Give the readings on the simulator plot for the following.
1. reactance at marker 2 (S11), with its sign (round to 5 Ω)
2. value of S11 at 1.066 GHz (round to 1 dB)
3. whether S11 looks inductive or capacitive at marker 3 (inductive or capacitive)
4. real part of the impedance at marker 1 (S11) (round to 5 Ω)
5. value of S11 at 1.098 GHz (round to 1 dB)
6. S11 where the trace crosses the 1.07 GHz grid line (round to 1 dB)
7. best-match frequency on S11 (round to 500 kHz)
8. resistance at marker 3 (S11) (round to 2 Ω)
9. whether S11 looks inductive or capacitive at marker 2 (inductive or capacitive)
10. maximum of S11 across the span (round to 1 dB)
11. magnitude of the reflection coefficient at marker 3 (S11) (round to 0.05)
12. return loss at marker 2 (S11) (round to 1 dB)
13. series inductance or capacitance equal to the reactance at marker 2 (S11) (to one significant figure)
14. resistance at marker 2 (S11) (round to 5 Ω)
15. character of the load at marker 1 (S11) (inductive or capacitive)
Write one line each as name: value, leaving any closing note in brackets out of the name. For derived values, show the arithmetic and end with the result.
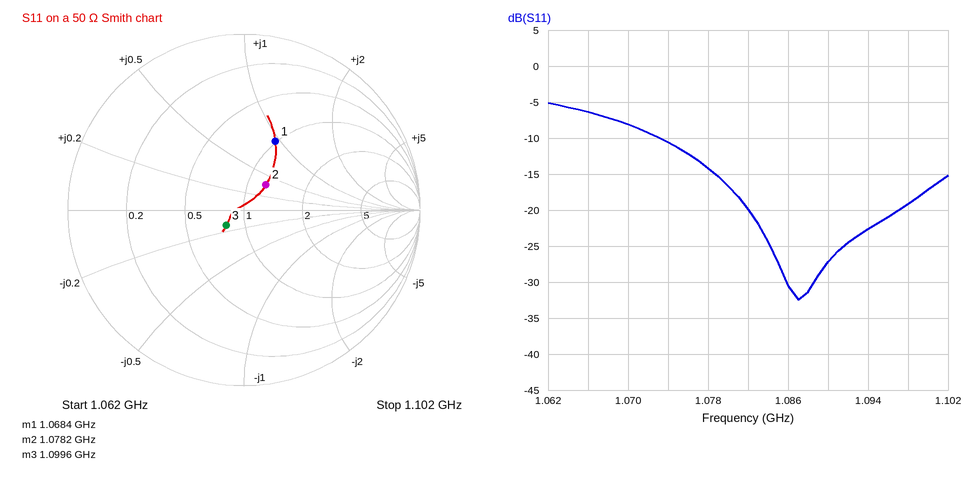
reactance at marker 2 (S11), with its sign: +20 Ω
value of S11 at 1.066 GHz: -6 dB
whether S11 looks inductive or capacitive at marker 3: capacitive
real part of the impedance at marker 1 (S11): 50 Ω
value of S11 at 1.098 GHz: -19 dB
S11 where the trace crosses the 1.07 GHz grid line: -8 dB
best-match frequency on S11: 1.0870 GHz
resistance at marker 3 (S11): 40 Ω
whether S11 looks inductive or capacitive at marker 2: inductive
maximum of S11 across the span: -5 dB
magnitude of the reflection coefficient at marker 3 (S11): 0.15
return loss at marker 2 (S11): 14 dB
series inductance or capacitance equal to the reactance at marker 2 (S11): L = 20 Ω/(2π × 1.0782 GHz) ≈ 3 nH
resistance at marker 2 (S11): 60 Ω
character of the load at marker 1 (S11): inductive
